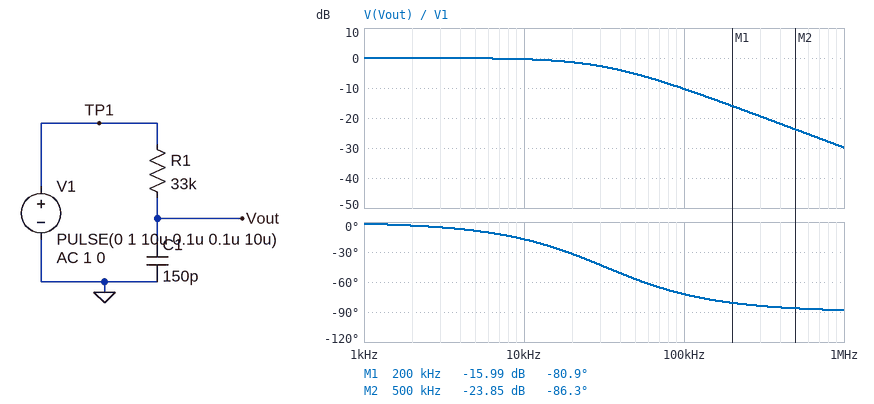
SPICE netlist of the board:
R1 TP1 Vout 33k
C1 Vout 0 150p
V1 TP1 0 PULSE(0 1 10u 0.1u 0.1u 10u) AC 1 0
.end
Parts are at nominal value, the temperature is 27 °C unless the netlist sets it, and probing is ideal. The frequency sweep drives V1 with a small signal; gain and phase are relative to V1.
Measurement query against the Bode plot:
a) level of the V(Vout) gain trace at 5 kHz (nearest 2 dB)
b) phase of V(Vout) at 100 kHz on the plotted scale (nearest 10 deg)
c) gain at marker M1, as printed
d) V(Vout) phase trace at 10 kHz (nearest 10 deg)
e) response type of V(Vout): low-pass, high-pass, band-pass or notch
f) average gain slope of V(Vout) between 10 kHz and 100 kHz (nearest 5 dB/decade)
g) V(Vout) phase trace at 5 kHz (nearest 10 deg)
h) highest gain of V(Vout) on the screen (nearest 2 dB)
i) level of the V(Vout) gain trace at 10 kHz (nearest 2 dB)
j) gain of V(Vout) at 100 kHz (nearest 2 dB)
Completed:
0 dB
-70 deg
-15.99 dB
-20 deg
low-pass
-10 dB/decade
-10 deg
0 dB
0 dB
-10 dB
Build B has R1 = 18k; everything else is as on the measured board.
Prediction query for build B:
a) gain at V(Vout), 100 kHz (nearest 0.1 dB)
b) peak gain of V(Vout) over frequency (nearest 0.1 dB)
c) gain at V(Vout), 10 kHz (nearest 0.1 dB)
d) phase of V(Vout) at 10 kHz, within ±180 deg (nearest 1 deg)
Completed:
-5.9 dB
0 dB
-0.1 dB
-10 deg
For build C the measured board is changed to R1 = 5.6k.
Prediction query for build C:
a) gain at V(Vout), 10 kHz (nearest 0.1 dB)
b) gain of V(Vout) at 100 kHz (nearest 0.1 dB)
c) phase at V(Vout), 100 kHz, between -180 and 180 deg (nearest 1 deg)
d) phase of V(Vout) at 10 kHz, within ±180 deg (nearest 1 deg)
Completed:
0 dB
-1.1 dB
-28 deg
-3 deg
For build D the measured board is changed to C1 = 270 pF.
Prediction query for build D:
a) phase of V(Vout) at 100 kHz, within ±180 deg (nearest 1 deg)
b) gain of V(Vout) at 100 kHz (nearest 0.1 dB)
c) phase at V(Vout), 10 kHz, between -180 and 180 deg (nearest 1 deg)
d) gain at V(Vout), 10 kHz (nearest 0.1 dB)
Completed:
-80 deg
-15.1 dB
-29 deg
-1.2 dB
